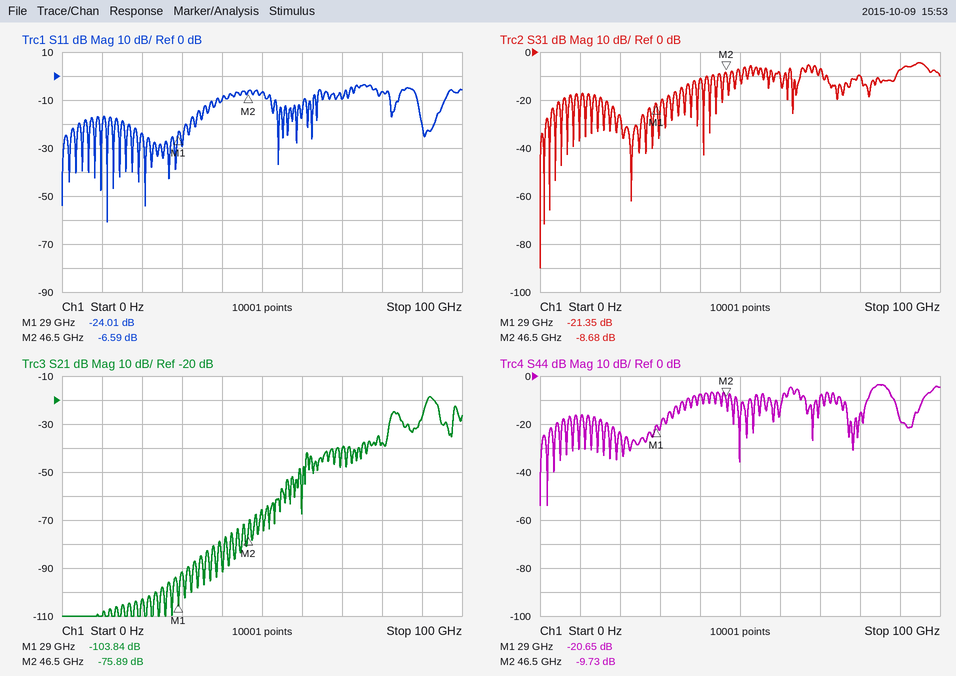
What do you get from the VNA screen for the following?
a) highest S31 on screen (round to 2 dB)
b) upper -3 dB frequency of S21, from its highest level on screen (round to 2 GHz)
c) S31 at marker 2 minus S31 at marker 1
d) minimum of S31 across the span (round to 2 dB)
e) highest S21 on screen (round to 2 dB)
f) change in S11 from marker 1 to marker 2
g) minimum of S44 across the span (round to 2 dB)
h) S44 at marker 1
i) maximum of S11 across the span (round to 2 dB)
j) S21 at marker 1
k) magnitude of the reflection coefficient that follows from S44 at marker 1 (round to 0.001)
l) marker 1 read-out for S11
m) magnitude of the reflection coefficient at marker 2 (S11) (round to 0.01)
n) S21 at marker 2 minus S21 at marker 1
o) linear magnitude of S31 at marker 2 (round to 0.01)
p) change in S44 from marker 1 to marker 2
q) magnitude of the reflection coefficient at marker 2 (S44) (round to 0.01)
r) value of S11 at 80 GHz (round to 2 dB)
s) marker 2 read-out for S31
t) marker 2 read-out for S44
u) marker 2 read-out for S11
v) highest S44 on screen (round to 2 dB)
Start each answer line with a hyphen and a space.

- -4 dB
- 94 GHz
- 12.67 dB
- -90 dB
- -18 dB
- 17.42 dB
- -54 dB
- -20.65 dB
- -4 dB
- -103.84 dB
- 0.093
- -24.01 dB
- 0.47
- 27.95 dB
- 0.37
- 10.92 dB
- 0.33
- -6 dB
- -8.68 dB
- -9.73 dB
- -6.59 dB
- -4 dB
